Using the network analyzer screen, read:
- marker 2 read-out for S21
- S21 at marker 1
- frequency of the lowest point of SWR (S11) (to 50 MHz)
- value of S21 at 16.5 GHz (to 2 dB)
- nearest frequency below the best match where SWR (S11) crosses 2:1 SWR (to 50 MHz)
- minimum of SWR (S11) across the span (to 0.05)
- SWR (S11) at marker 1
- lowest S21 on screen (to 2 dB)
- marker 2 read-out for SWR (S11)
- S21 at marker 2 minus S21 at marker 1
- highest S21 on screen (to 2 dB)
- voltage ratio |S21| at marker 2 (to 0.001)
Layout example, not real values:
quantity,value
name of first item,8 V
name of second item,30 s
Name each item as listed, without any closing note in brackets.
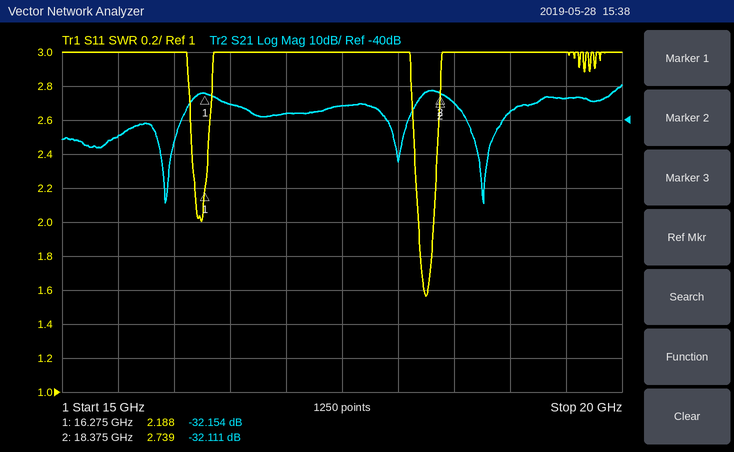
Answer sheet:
quantity,value
marker 2 read-out for S21,-32.111 dB
S21 at marker 1,-32.154 dB
frequency of the lowest point of SWR (S11),18.25 GHz
value of S21 at 16.5 GHz,-36 dB
nearest frequency below the best match where SWR (S11) crosses 2:1 SWR,18.20 GHz
minimum of SWR (S11) across the span,1.55
SWR (S11) at marker 1,2.188
lowest S21 on screen,-64 dB
marker 2 read-out for SWR,2.739
S21 at marker 2 minus S21 at marker 1,0.043 dB
highest S21 on screen,-30 dB
voltage ratio |S21| at marker 2,0.025
